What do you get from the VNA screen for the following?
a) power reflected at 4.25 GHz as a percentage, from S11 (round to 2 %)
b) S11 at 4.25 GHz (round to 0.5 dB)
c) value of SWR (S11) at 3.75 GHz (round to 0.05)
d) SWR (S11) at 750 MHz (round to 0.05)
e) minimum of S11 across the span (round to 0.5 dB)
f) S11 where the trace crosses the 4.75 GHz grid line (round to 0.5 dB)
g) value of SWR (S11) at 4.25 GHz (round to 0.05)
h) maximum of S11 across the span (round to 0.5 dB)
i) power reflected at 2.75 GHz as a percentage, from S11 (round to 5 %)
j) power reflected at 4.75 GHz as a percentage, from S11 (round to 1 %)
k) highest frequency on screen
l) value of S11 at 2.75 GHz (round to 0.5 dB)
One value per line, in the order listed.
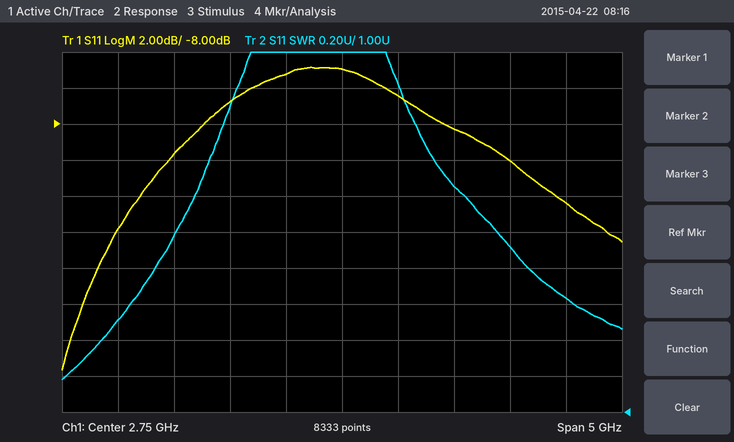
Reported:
10 %
-10.0 dB
2.25
1.50
-21.5 dB
-12.5 dB
1.90
-5.0 dB
30 %
6 %
5.25 GHz
-5.0 dB
